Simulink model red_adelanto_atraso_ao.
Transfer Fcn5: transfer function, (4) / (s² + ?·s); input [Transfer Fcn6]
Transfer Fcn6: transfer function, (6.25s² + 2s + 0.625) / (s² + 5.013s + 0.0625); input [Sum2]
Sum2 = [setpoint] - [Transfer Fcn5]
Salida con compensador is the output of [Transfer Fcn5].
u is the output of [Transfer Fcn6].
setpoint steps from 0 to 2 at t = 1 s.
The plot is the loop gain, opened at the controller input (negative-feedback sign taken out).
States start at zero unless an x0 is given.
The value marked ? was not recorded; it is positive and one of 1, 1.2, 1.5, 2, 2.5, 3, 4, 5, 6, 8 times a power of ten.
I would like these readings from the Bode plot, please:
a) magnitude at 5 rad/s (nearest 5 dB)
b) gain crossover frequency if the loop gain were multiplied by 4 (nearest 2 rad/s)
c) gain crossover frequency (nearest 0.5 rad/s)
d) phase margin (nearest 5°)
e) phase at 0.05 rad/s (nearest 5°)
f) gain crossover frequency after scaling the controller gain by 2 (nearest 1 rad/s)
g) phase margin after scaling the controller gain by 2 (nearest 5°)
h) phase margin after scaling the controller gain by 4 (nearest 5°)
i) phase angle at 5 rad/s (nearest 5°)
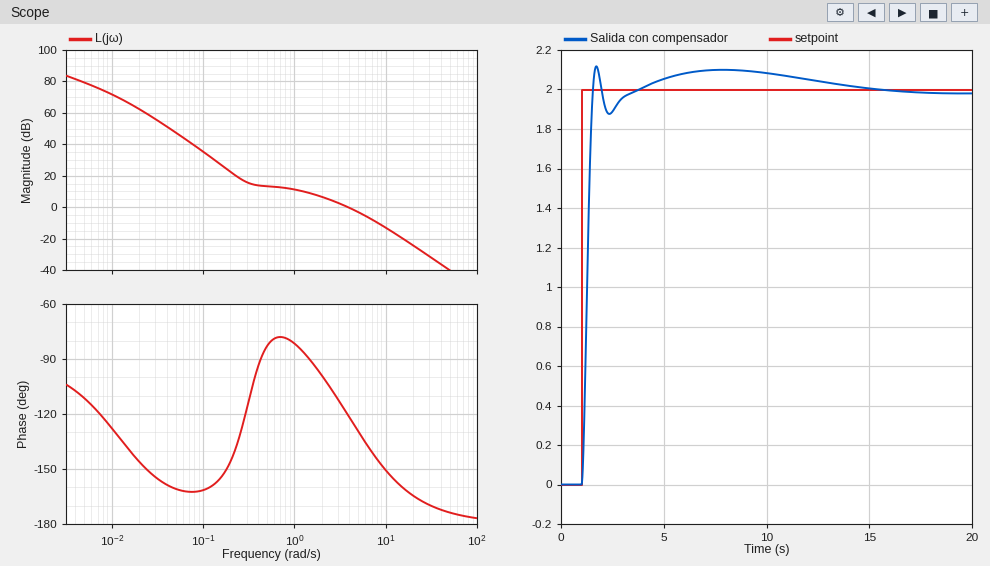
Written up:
-5 dB
10 rad/s
4.0 rad/s
60°
-160°
6 rad/s
45°
30°
-130°
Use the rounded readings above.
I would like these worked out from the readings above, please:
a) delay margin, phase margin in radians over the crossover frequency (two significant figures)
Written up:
0.26 s
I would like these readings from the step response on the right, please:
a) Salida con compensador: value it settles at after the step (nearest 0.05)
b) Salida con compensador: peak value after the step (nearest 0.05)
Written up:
2.00
2.10
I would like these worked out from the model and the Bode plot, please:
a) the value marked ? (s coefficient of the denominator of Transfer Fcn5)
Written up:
0.8
